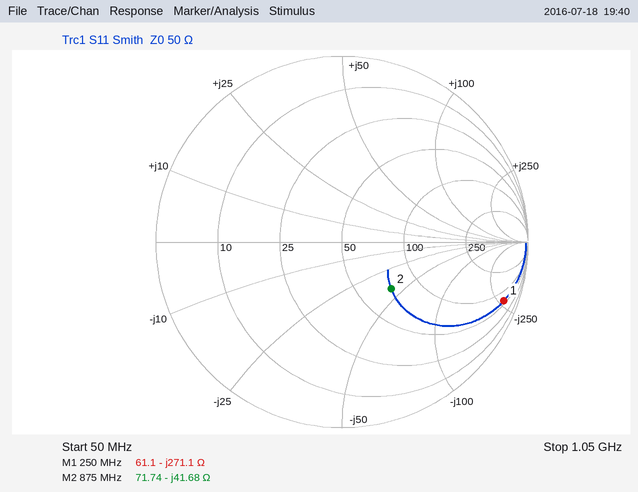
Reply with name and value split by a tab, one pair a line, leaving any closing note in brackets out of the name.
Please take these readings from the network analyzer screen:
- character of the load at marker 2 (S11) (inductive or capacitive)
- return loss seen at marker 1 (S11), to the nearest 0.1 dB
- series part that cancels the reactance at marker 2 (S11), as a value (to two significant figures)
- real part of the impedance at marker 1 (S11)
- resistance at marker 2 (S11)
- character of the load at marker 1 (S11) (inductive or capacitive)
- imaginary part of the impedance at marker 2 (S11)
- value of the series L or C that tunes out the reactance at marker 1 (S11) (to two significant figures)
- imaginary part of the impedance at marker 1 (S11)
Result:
character of the load at marker 2 (S11)	capacitive
return loss seen at marker 1 (S11), to the nearest 0.1 dB	0.7 dB
series part that cancels the reactance at marker 2 (S11), as a value	7.6 nH
real part of the impedance at marker 1	61.1 Ω
resistance at marker 2	71.74 Ω
character of the load at marker 1 (S11)	capacitive
imaginary part of the impedance at marker 2	-41.68 Ω
value of the series L or C that tunes out the reactance at marker 1 (S11)	170 nH
imaginary part of the impedance at marker 1	-271.1 Ω
